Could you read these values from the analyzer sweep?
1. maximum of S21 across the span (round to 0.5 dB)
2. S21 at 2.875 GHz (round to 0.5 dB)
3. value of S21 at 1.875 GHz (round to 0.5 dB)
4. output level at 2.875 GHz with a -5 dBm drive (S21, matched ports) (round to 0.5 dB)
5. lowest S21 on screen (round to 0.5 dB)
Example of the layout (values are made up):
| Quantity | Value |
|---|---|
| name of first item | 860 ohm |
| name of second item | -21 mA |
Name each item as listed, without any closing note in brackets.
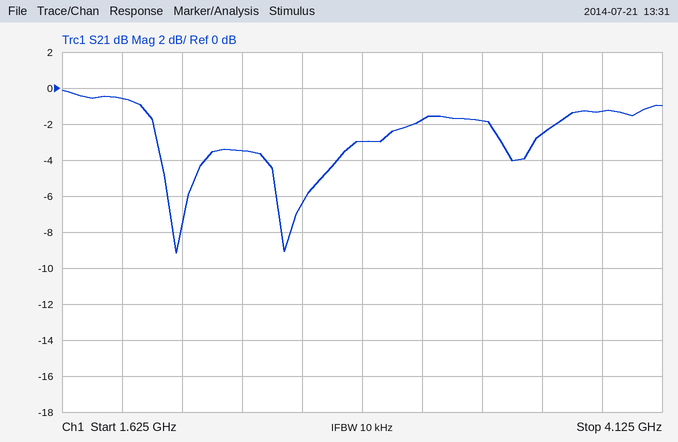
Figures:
| Quantity | Value |
|---|---|
| maximum of S21 across the span | 0.0 dB |
| S21 at 2.875 GHz | -3.0 dB |
| value of S21 at 1.875 GHz | -0.5 dB |
| output level at 2.875 GHz with a -5 dBm drive (S21, matched ports) | -8.0 dBm |
| lowest S21 on screen | -9.0 dB |
